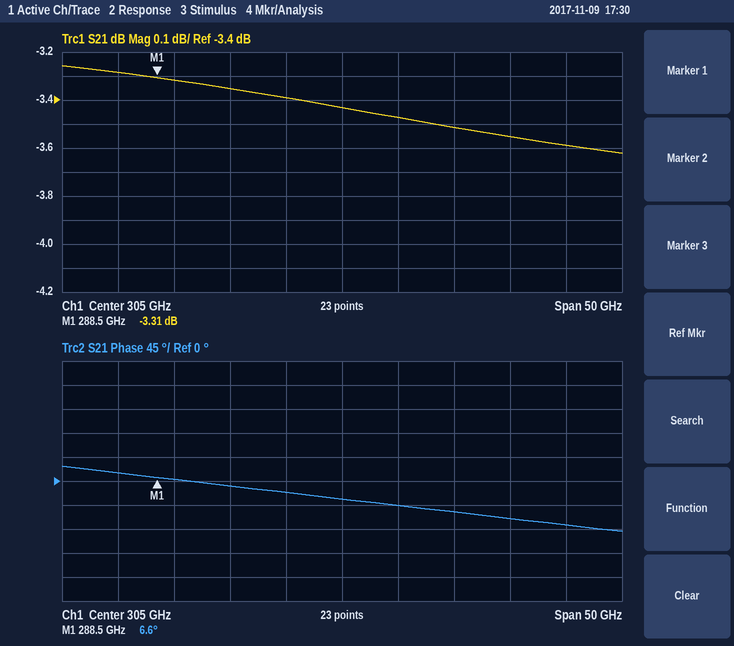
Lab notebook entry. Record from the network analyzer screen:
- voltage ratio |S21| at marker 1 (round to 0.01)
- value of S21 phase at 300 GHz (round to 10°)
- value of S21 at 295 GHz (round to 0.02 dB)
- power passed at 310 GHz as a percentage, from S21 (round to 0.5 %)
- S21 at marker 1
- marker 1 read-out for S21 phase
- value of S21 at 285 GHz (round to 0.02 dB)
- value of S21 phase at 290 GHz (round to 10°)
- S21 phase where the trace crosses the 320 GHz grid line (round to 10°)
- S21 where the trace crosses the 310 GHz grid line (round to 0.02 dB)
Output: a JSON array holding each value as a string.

["0.68", "-20°", "-3.36 dB", "45.0 %", "-3.31 dB", "6.6°", "-3.28 dB", "0°", "-70°", "-3.48 dB"]
